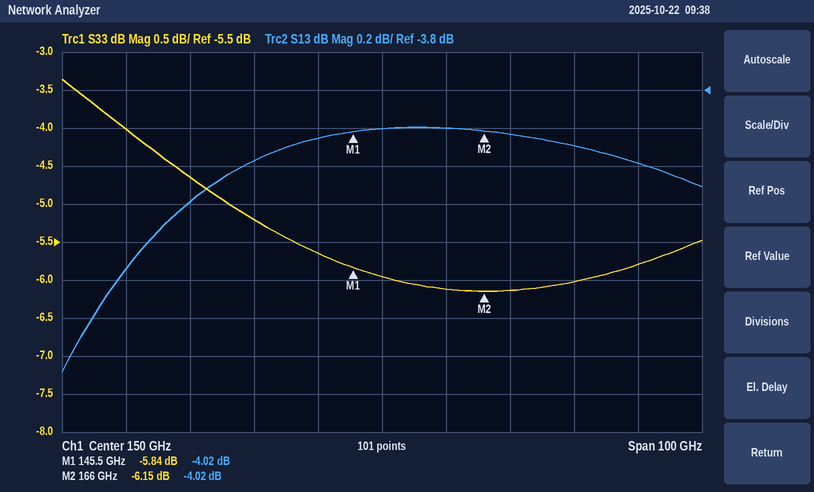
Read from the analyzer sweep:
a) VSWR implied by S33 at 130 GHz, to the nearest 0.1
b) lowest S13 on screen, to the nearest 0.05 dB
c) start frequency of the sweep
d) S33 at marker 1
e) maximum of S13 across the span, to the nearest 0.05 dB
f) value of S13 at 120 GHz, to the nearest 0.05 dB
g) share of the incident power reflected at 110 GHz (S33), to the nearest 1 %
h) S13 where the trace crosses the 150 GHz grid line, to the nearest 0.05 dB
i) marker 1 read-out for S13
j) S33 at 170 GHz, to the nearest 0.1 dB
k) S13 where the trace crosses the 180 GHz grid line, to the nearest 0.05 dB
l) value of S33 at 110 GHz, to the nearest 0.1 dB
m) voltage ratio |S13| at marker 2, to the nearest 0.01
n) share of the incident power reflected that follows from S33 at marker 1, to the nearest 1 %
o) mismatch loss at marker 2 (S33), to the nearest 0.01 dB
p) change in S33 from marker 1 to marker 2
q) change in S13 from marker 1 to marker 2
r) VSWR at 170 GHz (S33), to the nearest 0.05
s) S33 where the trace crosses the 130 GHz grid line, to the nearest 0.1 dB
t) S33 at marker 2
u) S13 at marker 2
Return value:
3.4
-5.30 dB
100 GHz
-5.84 dB
-4.00 dB
-4.40 dB
40 %
-4.00 dB
-4.02 dB
-6.1 dB
-4.10 dB
-4.0 dB
0.63
26 %
1.21 dB
-0.31 dB
0.00 dB
2.95
-5.2 dB
-6.15 dB
-4.02 dB
